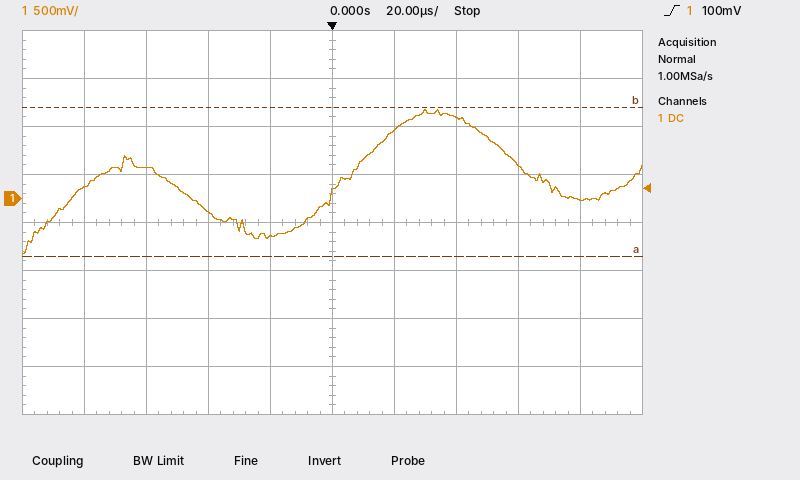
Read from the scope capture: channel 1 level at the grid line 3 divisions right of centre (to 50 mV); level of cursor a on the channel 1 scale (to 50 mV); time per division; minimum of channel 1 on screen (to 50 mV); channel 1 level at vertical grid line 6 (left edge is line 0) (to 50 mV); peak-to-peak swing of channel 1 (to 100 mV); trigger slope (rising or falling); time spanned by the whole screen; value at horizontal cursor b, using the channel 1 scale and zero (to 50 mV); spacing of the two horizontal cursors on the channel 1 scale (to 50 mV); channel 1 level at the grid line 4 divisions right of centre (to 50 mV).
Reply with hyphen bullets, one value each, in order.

- 350 mV
- -600 mV
- 20 µs
- -600 mV
- 700 mV
- 1.50 V
- rising
- 200 µs
- 950 mV
- 1.55 V
- 0 mV
